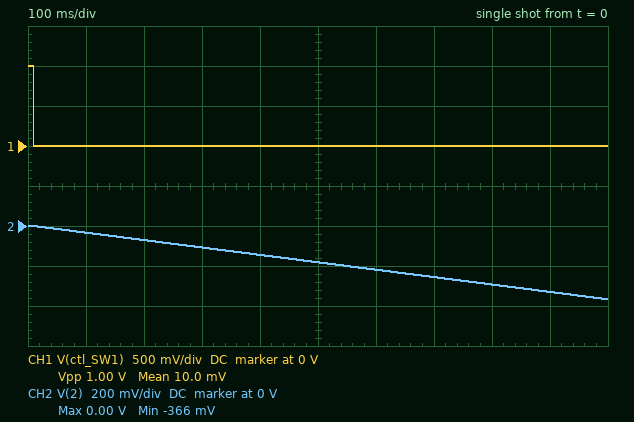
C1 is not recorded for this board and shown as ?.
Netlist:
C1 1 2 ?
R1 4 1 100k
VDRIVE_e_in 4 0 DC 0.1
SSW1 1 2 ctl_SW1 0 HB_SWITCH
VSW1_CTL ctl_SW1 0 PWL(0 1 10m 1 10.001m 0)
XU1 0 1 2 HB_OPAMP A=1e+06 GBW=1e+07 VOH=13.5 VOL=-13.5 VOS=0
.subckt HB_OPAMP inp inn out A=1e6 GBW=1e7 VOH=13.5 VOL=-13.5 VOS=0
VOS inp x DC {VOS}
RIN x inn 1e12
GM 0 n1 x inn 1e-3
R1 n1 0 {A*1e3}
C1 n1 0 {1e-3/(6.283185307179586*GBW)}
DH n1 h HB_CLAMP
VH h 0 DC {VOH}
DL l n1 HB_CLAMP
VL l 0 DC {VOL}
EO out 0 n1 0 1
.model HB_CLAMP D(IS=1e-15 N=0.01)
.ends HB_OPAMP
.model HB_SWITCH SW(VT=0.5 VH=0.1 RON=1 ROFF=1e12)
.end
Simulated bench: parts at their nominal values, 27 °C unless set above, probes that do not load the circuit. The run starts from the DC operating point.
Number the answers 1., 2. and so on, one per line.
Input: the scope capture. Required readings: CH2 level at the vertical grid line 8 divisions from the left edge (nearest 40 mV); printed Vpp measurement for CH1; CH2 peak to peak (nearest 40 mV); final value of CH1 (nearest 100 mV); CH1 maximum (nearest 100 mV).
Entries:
1. -280 mV
2. 1.00 V
3. 360 mV
4. 0 V
5. 1.0 V
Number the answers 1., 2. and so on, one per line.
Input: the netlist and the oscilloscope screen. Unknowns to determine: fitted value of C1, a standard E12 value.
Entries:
1. 2.7 µF
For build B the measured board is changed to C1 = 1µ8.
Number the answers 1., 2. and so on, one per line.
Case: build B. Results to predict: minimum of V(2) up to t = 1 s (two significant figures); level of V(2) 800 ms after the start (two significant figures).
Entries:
1. -550 mV
2. -440 mV
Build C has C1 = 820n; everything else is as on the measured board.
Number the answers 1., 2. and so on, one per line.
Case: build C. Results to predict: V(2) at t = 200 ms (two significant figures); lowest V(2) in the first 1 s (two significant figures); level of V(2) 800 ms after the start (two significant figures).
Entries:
1. -230 mV
2. -1.2 V
3. -960 mV
